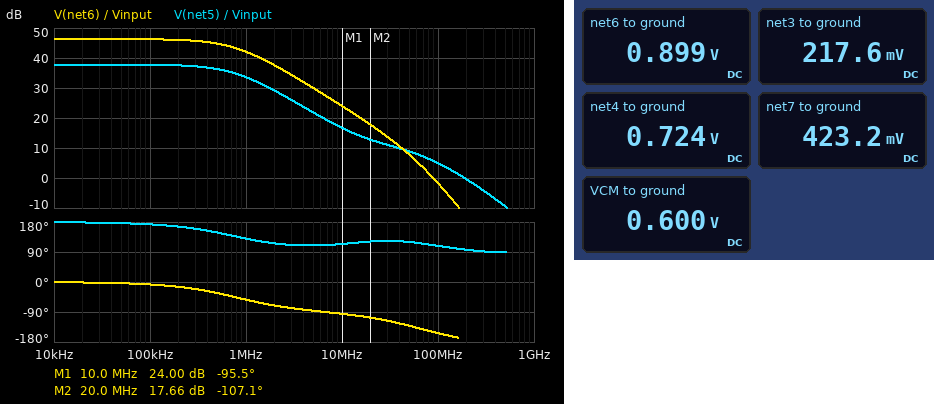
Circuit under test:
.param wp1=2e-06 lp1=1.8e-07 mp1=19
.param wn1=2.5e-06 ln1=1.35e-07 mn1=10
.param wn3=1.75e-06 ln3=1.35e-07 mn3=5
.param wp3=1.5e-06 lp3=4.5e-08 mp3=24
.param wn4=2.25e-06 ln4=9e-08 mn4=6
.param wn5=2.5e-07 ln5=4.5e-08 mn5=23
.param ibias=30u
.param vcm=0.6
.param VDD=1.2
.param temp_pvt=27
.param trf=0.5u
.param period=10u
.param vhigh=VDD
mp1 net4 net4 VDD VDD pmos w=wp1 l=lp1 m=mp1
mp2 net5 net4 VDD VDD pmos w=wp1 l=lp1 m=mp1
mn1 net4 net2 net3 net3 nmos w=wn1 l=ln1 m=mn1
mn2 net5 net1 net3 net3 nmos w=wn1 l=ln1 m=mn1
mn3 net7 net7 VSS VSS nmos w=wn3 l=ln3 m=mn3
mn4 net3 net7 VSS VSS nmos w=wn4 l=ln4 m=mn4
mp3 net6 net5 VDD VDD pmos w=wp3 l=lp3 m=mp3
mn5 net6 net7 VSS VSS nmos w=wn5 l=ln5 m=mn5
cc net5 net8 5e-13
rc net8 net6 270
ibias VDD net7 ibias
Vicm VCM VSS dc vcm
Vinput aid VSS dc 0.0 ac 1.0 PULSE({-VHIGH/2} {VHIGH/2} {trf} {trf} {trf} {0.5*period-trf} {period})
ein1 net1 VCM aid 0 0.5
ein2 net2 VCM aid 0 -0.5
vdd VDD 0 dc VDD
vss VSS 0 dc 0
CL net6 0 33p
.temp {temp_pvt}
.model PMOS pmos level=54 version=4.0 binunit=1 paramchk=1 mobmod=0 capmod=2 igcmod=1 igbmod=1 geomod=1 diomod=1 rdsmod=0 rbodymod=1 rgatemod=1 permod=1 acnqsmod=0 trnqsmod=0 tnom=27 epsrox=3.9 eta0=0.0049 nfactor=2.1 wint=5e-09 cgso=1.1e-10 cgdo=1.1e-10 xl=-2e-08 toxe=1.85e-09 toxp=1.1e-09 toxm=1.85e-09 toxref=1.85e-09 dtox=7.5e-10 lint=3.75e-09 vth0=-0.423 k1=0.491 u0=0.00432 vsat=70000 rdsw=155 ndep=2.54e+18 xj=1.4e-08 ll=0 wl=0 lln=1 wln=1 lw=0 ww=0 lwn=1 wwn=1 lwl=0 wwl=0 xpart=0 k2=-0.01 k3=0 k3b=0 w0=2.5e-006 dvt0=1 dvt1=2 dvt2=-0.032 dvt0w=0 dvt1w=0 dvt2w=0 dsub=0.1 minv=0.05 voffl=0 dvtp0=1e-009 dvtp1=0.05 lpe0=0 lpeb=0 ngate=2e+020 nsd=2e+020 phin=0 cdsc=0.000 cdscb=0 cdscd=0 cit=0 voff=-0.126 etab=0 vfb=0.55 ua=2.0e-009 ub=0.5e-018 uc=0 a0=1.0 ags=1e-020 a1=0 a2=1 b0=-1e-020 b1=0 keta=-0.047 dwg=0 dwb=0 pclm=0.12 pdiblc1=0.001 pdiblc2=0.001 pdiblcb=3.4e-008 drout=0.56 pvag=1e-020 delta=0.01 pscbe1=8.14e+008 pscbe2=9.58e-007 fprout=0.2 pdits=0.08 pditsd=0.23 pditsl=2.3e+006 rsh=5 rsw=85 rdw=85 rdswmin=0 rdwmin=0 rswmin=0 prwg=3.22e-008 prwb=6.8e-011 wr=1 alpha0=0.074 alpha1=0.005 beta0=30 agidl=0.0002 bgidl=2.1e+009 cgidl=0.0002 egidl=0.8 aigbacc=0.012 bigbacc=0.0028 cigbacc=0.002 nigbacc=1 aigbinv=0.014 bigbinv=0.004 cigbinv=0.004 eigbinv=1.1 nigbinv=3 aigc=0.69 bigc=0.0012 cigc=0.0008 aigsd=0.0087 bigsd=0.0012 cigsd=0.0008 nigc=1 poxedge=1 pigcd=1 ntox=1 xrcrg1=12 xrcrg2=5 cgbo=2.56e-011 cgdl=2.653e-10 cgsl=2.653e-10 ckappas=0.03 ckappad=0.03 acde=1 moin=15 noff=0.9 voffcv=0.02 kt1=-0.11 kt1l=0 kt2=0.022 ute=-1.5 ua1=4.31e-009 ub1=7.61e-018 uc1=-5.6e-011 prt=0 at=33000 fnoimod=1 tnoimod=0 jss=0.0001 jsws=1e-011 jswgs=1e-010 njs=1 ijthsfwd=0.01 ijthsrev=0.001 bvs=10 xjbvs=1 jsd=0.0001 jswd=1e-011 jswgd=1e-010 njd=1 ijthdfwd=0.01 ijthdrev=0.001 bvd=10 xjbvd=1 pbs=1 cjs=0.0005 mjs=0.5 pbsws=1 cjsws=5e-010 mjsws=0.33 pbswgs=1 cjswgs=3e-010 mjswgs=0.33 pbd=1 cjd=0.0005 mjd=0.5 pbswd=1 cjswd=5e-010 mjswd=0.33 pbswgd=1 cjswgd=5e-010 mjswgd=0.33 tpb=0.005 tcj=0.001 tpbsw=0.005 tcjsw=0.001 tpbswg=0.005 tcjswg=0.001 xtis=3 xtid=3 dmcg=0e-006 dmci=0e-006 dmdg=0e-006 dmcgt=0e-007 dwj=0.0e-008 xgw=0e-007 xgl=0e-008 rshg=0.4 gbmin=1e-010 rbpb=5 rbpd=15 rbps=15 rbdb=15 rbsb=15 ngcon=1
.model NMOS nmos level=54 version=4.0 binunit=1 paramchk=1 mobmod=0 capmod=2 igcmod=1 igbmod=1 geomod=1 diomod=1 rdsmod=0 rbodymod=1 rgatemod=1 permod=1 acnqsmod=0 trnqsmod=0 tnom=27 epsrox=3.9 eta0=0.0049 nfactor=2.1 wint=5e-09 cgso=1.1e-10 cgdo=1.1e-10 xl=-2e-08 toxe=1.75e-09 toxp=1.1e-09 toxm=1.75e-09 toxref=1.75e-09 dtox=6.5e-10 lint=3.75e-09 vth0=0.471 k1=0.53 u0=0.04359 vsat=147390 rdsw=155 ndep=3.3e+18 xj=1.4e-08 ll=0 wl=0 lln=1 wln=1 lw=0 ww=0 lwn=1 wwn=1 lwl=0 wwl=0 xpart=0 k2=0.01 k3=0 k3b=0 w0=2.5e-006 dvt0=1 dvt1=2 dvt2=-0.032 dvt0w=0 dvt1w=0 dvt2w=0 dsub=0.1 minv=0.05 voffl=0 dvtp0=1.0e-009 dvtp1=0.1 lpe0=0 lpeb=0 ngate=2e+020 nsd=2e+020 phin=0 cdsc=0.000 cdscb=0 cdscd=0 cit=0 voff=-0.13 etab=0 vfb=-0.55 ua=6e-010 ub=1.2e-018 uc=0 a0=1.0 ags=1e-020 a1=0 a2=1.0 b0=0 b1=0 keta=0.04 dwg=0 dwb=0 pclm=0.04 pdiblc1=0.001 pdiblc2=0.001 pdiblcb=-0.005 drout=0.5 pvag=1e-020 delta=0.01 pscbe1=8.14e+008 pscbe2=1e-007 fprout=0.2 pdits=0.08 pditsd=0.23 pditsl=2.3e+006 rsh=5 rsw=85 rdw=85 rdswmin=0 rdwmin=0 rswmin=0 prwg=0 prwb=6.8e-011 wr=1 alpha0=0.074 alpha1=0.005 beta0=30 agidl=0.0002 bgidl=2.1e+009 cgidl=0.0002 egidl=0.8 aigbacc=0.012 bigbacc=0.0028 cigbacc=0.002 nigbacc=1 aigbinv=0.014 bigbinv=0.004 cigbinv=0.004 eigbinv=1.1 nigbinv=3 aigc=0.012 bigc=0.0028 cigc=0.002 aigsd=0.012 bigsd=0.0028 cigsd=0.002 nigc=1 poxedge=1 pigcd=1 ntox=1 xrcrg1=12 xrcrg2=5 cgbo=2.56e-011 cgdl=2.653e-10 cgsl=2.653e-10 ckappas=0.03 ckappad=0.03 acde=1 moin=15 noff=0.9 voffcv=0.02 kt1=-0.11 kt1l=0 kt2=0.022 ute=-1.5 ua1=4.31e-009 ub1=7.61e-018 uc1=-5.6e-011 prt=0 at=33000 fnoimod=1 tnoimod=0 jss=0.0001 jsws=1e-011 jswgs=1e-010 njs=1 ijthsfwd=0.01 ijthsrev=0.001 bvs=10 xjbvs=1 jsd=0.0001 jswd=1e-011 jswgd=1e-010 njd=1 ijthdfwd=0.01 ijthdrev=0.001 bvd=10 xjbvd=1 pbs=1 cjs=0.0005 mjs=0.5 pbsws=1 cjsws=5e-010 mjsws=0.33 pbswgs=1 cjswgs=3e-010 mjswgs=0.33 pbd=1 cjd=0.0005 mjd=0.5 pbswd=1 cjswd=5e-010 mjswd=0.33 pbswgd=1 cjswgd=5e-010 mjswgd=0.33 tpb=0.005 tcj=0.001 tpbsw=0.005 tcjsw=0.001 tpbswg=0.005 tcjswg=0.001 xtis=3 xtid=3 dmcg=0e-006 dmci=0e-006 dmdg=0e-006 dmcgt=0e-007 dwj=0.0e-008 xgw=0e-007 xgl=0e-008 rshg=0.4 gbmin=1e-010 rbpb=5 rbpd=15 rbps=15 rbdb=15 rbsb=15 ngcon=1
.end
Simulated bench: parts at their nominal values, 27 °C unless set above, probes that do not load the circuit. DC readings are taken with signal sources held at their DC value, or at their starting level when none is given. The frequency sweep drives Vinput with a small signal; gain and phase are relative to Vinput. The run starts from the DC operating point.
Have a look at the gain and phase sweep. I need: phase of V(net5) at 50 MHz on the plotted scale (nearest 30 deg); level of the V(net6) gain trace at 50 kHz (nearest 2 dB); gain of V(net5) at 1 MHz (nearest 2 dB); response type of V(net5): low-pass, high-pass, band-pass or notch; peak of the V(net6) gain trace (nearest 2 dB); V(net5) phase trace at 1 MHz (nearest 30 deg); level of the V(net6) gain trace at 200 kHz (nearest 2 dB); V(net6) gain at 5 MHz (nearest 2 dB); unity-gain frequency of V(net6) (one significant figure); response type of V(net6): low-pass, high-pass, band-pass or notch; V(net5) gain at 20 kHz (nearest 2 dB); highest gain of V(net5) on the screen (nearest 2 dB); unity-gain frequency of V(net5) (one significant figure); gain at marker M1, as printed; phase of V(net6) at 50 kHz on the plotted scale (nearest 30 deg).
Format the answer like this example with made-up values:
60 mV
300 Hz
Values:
120 deg
46 dB
34 dB
low-pass
46 dB
120 deg
46 dB
30 dB
90 MHz
low-pass
38 dB
38 dB
200 MHz
24.00 dB
0 deg
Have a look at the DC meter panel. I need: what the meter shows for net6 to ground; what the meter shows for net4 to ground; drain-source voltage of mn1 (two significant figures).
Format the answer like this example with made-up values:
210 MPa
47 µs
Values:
0.899 V
0.724 V
510 mV
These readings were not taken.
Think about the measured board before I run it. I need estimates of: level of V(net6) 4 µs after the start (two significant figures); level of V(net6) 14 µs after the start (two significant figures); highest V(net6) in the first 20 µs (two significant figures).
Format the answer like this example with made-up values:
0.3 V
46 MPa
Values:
1.2 V
1.2 V
1.2 V
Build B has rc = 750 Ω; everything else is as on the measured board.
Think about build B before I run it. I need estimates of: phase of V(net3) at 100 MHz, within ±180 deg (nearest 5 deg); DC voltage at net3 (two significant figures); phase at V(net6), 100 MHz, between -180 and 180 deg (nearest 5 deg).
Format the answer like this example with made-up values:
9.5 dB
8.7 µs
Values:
140 deg
220 mV
-145 deg
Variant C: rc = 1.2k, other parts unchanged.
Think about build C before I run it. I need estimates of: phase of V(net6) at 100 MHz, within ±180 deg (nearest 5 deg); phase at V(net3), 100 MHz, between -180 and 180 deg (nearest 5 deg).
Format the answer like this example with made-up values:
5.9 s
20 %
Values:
-140 deg
150 deg
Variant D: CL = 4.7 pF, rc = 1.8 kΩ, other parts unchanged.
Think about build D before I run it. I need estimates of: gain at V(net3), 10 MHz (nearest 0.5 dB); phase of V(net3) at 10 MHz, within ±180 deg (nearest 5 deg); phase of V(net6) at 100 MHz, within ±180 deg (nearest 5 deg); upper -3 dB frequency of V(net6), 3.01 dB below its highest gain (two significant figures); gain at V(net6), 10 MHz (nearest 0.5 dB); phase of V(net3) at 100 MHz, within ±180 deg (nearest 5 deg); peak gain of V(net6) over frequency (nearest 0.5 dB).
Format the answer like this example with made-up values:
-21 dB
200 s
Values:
-32.5 dB
105 deg
-85 deg
800 kHz
24.5 dB
160 deg
46.5 dB
